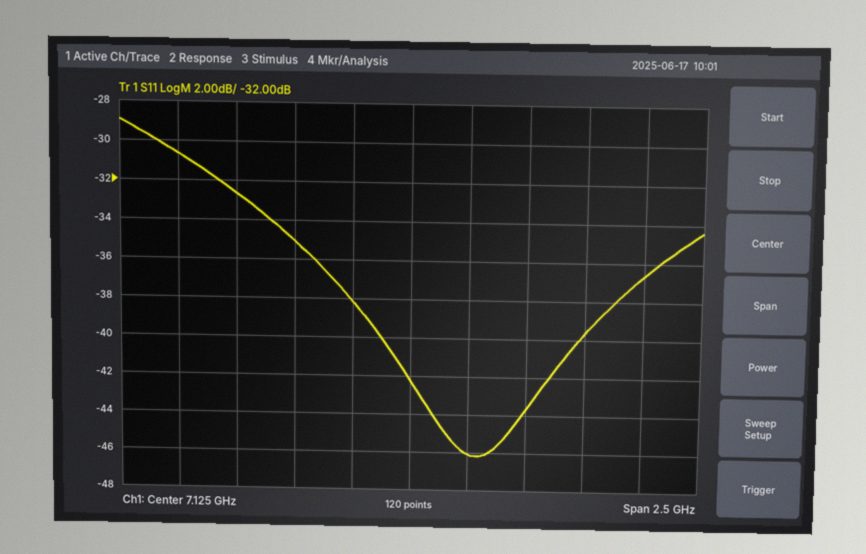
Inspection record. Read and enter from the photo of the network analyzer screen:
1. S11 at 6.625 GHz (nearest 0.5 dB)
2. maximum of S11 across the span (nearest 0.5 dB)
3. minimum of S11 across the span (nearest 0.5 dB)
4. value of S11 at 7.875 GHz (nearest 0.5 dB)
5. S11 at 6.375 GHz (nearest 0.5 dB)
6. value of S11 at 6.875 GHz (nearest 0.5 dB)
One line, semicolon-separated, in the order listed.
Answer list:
-35.0 dB; -29.0 dB; -46.0 dB; -39.5 dB; -32.5 dB; -38.0 dB
